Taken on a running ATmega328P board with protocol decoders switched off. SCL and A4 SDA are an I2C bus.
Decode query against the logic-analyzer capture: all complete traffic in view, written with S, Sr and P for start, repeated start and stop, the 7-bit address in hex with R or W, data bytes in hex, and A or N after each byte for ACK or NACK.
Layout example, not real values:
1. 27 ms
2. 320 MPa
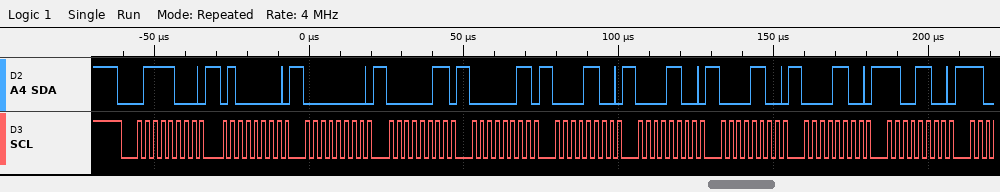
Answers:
1. S 3CW A 40 A 00 A 03 A 03 A 0C A 0C A 0C A 0C A CC A
